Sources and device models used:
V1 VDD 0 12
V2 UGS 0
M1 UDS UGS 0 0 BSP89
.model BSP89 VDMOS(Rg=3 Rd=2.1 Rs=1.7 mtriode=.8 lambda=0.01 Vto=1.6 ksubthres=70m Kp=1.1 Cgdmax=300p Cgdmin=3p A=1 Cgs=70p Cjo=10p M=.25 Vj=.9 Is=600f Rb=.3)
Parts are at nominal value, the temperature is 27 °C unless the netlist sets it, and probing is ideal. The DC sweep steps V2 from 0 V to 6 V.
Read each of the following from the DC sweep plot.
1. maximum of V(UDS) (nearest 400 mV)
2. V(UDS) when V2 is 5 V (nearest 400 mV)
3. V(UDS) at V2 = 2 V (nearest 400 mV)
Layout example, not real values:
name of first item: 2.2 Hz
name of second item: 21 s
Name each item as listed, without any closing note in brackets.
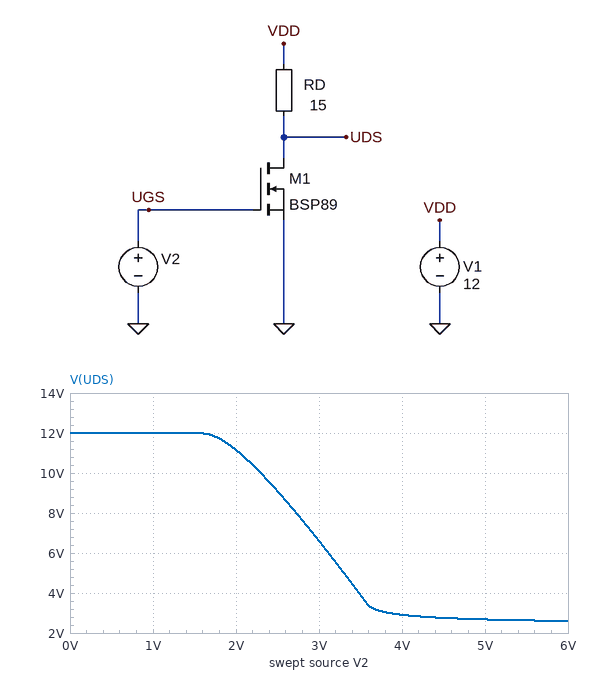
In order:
maximum of V(UDS): 12.0 V
V(UDS) when V2 is 5 V: 2.8 V
V(UDS) at V2 = 2 V: 11.2 V
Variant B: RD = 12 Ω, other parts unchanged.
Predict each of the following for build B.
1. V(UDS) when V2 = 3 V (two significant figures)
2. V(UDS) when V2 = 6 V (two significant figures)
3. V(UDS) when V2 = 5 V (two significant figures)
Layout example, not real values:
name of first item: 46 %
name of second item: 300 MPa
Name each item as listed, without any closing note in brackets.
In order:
V(UDS) when V2 = 3 V: 7.7 V
V(UDS) when V2 = 6 V: 3.1 V
V(UDS) when V2 = 5 V: 3.2 V
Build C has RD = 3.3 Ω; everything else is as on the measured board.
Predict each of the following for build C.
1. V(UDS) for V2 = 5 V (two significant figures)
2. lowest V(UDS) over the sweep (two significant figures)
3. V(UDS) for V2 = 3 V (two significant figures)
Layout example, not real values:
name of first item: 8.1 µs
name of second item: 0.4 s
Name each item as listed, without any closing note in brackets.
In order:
V(UDS) for V2 = 5 V: 8.2 V
lowest V(UDS) over the sweep: 7.0 V
V(UDS) for V2 = 3 V: 11 V
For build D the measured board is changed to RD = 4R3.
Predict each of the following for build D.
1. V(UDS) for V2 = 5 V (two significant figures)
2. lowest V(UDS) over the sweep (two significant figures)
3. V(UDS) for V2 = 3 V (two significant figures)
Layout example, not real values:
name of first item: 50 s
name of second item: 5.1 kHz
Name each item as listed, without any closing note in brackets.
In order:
V(UDS) for V2 = 5 V: 7.0 V
lowest V(UDS) over the sweep: 6.1 V
V(UDS) for V2 = 3 V: 10 V
